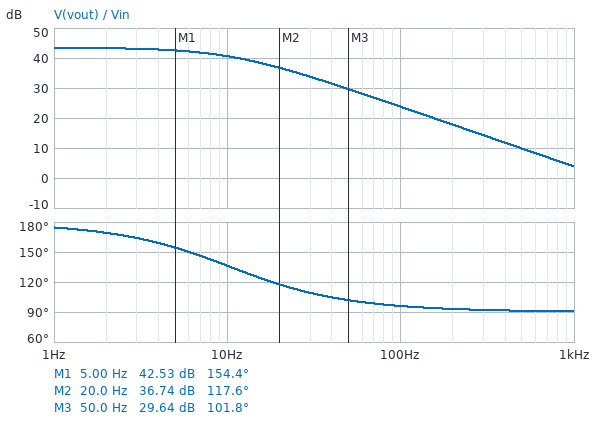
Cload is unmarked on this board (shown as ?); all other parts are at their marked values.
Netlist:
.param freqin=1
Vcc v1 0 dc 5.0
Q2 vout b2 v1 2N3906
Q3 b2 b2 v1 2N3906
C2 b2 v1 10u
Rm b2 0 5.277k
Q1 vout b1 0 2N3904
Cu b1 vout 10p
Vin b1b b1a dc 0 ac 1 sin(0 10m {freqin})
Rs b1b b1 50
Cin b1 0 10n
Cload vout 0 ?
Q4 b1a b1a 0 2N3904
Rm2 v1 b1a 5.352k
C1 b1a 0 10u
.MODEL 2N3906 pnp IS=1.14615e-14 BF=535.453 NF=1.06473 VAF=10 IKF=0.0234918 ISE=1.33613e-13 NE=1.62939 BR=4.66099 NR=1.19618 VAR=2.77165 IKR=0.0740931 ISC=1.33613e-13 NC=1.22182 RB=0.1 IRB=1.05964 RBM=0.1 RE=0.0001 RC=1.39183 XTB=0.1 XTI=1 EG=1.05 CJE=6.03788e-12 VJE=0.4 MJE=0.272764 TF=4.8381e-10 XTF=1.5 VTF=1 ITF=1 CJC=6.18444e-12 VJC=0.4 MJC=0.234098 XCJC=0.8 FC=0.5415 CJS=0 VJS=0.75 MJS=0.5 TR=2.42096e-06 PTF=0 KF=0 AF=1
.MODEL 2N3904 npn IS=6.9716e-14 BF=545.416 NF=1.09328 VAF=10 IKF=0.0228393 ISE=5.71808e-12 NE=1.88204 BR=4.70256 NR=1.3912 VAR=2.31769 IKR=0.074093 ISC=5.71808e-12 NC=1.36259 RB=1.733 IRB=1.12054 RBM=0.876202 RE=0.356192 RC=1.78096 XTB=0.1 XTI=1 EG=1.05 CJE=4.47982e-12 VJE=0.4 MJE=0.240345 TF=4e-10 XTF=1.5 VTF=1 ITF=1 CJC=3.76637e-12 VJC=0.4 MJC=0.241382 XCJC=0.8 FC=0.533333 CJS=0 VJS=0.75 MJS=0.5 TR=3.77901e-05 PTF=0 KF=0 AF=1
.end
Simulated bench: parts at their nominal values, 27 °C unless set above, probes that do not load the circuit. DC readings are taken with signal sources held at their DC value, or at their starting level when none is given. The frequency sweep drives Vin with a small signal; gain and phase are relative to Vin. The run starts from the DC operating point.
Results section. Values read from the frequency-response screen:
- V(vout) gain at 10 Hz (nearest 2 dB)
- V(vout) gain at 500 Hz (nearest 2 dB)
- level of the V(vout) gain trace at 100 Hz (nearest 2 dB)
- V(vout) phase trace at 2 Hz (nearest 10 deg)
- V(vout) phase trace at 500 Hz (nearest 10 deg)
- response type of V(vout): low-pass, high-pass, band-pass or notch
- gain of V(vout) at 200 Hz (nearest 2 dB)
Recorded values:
40 dB
10 dB
24 dB
170 deg
90 deg
low-pass
18 dB
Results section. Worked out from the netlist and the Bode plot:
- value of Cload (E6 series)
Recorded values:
3.3 µF
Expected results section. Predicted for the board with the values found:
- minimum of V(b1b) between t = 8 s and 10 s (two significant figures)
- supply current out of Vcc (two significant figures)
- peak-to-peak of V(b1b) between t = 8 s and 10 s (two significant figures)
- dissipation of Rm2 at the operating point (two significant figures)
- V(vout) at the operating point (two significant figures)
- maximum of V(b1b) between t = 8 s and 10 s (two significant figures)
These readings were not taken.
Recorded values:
660 mV
2.6 mA
20 mV
3.5 mW
2.6 V
680 mV
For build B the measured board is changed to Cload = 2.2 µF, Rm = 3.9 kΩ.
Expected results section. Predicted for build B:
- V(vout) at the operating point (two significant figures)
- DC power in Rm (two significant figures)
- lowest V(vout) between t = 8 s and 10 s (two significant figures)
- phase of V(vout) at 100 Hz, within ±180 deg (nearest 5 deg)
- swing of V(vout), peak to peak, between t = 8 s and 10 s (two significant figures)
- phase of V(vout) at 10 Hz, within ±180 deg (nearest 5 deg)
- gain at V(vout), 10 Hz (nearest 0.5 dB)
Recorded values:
3.9 V
4.7 mW
2.5 V
100 deg
2.4 V
150 deg
42.0 dB
